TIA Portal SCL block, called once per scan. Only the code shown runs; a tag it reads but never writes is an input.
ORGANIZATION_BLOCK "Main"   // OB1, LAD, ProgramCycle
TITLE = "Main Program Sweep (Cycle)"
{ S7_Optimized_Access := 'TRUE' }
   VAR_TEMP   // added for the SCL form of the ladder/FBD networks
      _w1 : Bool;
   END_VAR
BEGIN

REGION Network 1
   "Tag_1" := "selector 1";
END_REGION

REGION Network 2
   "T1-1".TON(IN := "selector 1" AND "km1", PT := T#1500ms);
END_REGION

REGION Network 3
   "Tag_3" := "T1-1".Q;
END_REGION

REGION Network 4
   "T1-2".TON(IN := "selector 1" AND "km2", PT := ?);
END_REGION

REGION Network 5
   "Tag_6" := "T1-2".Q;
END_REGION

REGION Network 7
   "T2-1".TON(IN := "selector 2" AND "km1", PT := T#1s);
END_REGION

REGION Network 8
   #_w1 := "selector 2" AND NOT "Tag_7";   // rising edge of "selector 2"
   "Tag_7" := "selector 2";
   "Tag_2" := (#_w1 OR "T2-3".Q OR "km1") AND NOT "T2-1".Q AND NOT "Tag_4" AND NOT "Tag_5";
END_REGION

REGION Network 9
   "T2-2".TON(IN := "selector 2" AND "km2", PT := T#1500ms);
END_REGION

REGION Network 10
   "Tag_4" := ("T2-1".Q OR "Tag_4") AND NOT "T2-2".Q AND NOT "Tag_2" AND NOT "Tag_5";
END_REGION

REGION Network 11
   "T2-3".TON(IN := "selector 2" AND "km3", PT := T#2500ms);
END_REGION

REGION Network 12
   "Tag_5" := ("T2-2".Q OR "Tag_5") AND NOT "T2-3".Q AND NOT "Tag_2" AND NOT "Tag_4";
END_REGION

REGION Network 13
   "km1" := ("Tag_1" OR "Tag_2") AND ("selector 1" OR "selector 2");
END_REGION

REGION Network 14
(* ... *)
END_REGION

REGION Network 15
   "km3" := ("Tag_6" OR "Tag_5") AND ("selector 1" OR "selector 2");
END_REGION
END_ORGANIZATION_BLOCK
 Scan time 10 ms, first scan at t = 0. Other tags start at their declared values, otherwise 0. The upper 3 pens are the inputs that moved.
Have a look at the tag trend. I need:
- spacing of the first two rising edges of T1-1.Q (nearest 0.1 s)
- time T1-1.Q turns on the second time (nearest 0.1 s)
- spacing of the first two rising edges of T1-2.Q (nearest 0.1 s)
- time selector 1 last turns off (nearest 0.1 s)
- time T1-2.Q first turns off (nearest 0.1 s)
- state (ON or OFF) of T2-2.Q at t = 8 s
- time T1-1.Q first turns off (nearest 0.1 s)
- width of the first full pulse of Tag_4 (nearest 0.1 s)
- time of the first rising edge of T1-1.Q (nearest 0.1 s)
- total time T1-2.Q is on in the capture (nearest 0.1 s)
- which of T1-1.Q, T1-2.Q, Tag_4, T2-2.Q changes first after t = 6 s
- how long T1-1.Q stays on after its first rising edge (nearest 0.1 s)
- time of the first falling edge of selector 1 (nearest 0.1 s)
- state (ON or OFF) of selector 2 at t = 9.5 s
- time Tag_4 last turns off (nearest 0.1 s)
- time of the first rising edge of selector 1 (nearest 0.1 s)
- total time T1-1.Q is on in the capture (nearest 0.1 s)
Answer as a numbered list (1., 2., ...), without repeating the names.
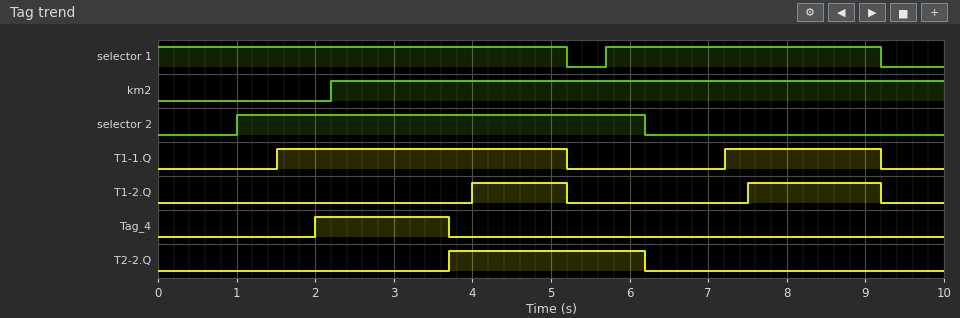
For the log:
1. 5.7 s
2. 7.2 s
3. 3.5 s
4. 9.2 s
5. 5.2 s
6. OFF
7. 5.2 s
8. 1.7 s
9. 1.5 s
10. 2.9 s
11. T2-2.Q
12. 3.7 s
13. 5.2 s
14. OFF
15. 3.7 s
16. 5.7 s
17. 5.7 s
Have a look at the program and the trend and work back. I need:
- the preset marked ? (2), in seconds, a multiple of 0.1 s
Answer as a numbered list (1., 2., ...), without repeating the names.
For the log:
1. 1.8 s
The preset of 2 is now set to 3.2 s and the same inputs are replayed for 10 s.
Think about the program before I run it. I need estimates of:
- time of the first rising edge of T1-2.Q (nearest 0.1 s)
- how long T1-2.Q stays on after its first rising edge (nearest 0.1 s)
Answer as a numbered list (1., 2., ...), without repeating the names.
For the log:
1. 8.9 s
2. 0.3 s
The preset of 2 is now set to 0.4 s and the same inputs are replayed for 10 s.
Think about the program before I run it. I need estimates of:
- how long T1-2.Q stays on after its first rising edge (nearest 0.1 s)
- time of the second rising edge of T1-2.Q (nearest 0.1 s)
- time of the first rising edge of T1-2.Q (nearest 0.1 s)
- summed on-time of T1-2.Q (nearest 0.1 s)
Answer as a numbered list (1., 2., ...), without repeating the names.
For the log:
1. 2.6 s
2. 6.1 s
3. 2.6 s
4. 5.7 s
